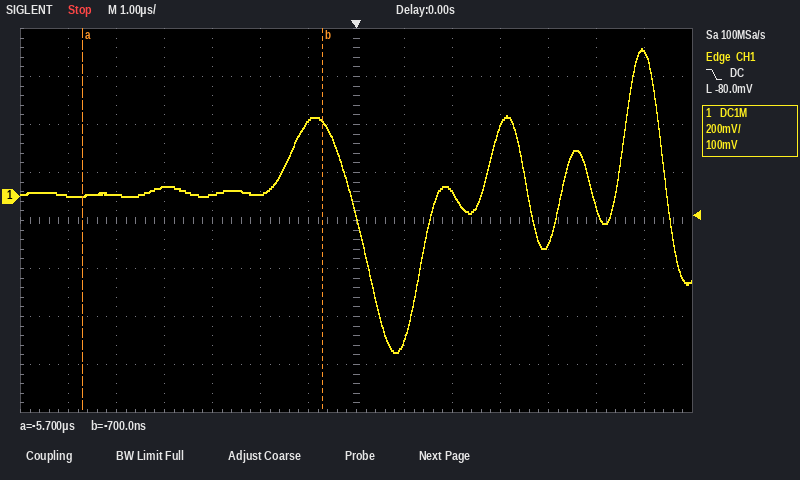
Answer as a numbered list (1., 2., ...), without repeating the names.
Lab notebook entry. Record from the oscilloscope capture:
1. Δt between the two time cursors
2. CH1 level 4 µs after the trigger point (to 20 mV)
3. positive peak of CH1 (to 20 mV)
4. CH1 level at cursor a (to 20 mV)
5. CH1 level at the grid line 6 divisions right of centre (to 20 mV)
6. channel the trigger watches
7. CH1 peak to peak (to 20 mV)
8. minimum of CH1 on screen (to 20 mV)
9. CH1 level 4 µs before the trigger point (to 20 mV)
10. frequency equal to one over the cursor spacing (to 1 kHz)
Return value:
1. 5.0 µs
2. -200 mV
3. 620 mV
4. 0 mV
5. 600 mV
6. CH1
7. 1.26 V
8. -640 mV
9. 40 mV
10. 200 kHz
